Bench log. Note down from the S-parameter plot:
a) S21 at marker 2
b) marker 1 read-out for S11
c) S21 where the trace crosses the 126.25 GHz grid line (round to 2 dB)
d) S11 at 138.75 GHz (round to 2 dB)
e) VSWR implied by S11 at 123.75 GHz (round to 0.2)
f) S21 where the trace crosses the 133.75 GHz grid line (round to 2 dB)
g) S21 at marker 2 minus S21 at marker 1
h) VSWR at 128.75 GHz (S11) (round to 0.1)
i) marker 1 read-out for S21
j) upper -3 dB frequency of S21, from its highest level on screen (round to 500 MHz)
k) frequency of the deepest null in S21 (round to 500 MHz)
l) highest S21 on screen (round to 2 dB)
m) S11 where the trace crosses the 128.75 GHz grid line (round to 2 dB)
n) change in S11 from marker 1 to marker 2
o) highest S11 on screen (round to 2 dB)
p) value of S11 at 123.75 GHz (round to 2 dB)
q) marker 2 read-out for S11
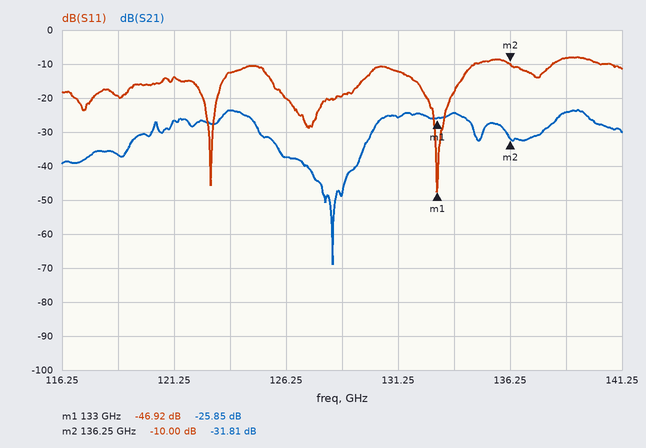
-31.81 dB
-46.92 dB
-38 dB
-8 dB
1.6
-24 dB
-5.96 dB
1.2
-25.85 dB
140.0 GHz
128.5 GHz
-24 dB
-20 dB
36.92 dB
-8 dB
-12 dB
-10.00 dB
